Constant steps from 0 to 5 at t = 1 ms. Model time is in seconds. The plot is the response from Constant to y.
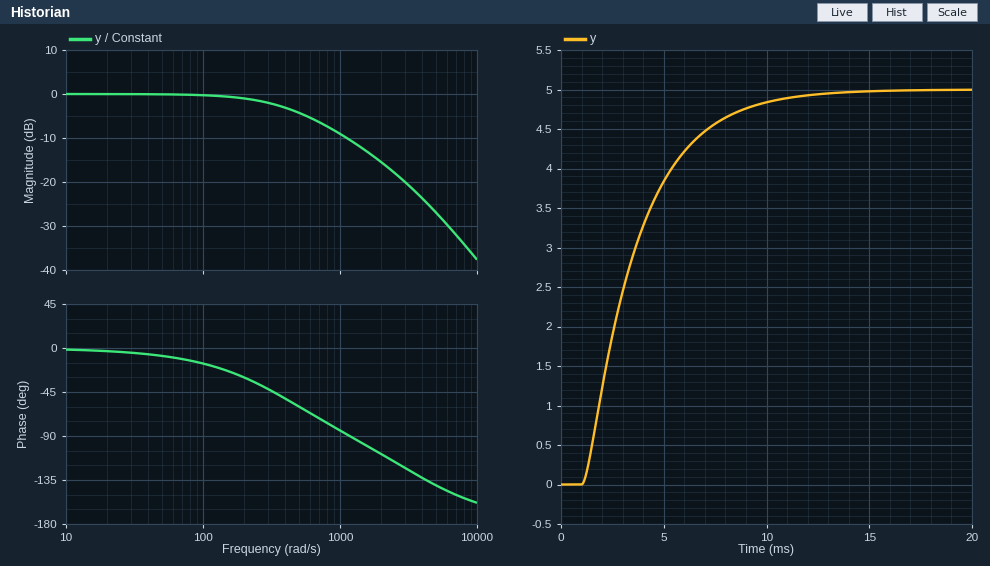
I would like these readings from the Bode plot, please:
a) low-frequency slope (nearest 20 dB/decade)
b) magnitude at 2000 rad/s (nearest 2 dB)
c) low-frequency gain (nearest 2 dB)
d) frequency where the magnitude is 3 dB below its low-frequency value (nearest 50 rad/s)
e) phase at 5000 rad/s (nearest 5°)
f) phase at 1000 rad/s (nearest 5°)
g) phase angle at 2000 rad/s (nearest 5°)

0 dB/decade
-16 dB
0 dB
400 rad/s
-140°
-85°
-110°
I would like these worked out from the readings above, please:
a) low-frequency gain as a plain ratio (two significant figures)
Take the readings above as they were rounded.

1.0
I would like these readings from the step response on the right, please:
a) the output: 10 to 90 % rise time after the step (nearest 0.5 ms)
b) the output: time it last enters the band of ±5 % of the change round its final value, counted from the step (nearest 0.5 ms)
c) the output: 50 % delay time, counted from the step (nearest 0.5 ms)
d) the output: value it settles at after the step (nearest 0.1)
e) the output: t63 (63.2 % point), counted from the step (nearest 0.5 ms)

5.5 ms
8.0 ms
2.0 ms
5.0
3.0 ms
